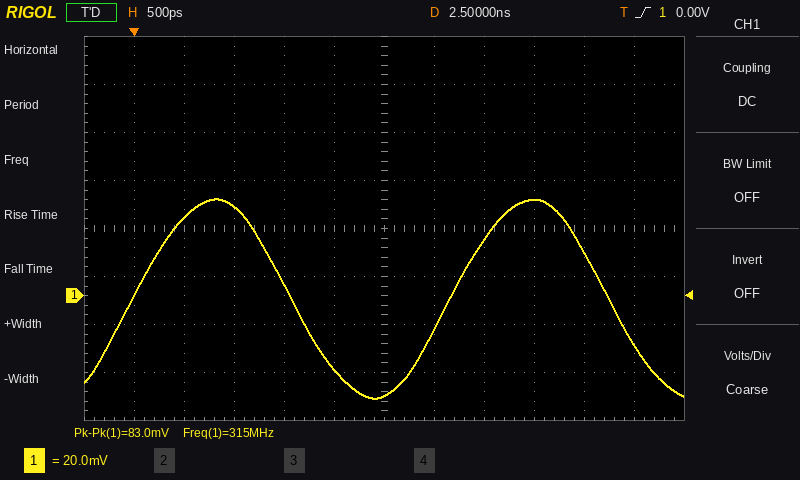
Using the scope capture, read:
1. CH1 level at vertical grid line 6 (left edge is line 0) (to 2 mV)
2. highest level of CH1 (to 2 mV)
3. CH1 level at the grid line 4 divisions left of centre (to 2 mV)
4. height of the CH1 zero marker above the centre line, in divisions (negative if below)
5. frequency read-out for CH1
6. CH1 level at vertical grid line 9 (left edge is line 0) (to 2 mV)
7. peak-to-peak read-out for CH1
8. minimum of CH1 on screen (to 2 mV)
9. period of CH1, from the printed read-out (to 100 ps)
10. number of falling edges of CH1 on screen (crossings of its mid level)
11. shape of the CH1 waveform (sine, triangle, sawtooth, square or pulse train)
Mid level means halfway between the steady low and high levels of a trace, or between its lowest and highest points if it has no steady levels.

-42 mV
40 mV
32 mV
-1.4 div
315 MHz
40 mV
83.0 mV
-42 mV
3.2 ns
2
sine
